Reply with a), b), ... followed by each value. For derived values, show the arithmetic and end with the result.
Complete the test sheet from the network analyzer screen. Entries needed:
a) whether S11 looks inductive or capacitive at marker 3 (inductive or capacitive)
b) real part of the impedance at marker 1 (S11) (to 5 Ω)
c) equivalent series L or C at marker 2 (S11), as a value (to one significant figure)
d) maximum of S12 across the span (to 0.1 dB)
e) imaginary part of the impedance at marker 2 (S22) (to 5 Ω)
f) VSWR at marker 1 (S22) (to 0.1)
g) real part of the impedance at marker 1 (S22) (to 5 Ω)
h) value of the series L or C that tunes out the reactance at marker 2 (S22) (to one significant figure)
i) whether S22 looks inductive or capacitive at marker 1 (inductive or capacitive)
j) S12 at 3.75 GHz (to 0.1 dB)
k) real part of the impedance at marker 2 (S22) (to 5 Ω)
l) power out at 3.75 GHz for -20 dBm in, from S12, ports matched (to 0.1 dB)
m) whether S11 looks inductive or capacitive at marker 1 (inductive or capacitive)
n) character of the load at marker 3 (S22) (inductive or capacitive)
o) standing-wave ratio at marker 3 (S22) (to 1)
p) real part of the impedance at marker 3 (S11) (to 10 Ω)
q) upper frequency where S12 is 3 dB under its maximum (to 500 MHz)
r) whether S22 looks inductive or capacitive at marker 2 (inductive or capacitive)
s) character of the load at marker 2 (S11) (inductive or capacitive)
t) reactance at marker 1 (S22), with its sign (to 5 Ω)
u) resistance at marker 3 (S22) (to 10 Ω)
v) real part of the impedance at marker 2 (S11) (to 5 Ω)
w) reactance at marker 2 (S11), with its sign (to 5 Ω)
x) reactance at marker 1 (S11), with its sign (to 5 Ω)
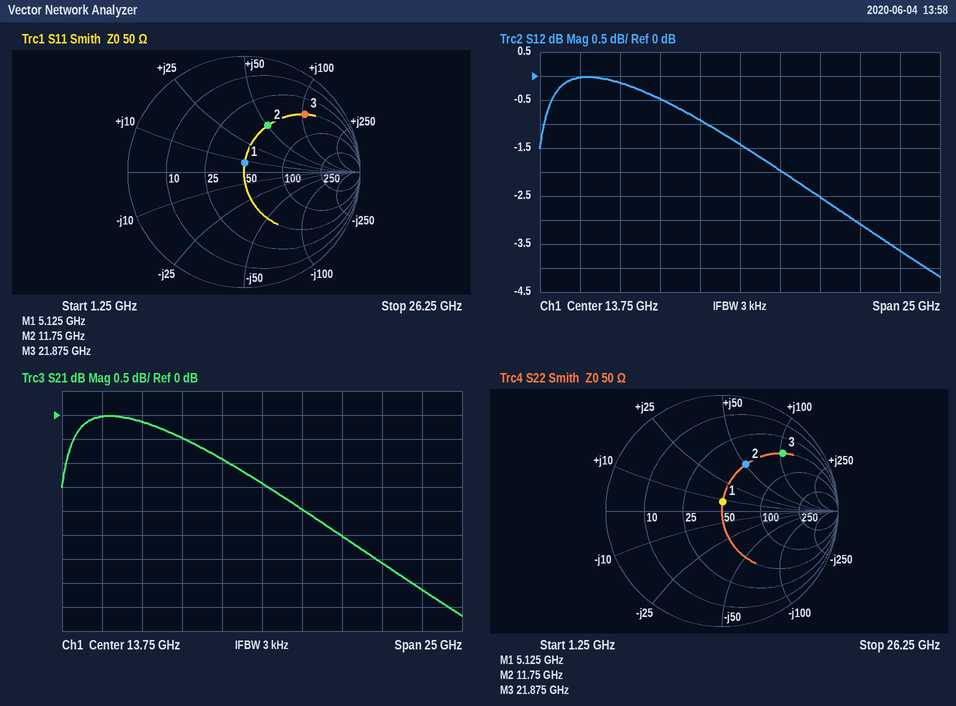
a) inductive
b) 50 Ω
c) L = 50 Ω/(2π × 11.75 GHz) ≈ 677 pH, so 700 pH to one significant figure
d) 0.0 dB
e) +50 Ω
f) 1.2
g) 50 Ω
h) C = 1/(2π × 11.75 GHz × 50 Ω) ≈ 271 fF, so 300 fF to one significant figure
i) inductive
j) 0.0 dB
k) 50 Ω
l) -20 dBm + (0.0 dB) = -20.0 dBm
m) inductive
n) inductive
o) 6
p) 50 Ω
q) 21.0 GHz
r) inductive
s) inductive
t) +10 Ω
u) 50 Ω
v) 50 Ω
w) +50 Ω
x) +10 Ω
